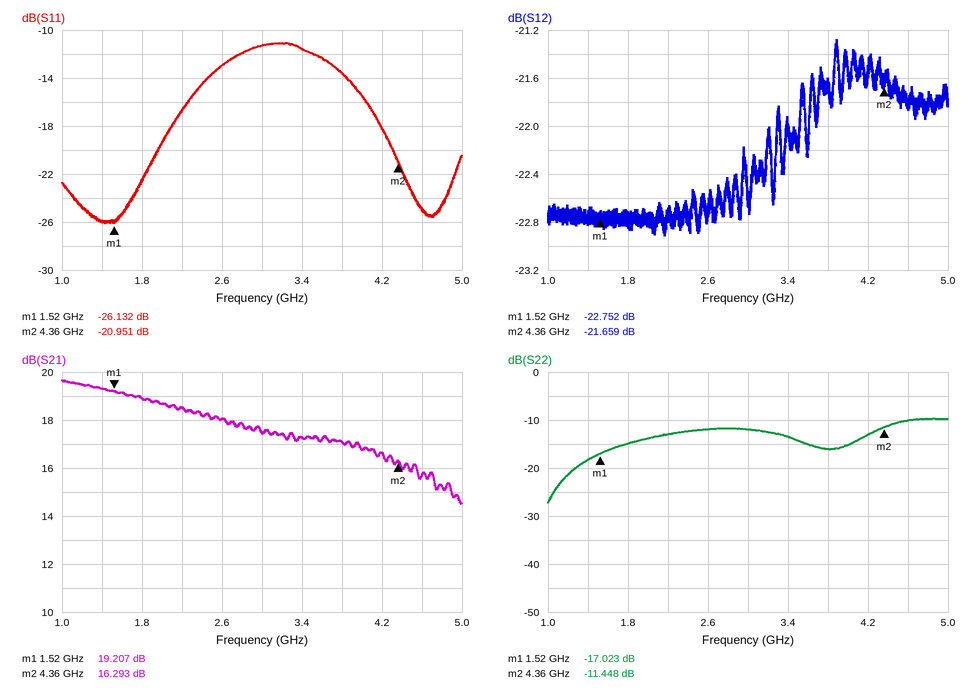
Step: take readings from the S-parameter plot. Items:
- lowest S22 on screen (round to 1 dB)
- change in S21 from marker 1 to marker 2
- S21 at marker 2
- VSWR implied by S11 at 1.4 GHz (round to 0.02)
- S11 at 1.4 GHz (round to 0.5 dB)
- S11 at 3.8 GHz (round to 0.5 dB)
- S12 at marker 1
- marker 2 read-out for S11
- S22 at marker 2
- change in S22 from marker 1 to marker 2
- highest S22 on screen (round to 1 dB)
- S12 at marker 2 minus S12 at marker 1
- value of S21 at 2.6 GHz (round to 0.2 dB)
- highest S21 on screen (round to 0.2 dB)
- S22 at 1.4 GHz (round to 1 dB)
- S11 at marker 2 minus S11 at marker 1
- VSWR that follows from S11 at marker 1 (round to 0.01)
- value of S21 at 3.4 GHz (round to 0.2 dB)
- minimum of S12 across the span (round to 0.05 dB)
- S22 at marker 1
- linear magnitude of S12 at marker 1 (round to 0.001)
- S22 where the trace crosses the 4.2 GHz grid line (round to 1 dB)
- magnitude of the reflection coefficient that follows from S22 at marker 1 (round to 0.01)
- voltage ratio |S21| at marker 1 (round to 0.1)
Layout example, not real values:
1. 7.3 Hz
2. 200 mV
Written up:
1. -27 dB
2. -2.914 dB
3. 16.293 dB
4. 1.10
5. -26.0 dB
6. -13.5 dB
7. -22.752 dB
8. -20.951 dB
9. -11.448 dB
10. 5.575 dB
11. -10 dB
12. 1.093 dB
13. 18.0 dB
14. 19.6 dB
15. -18 dB
16. 5.181 dB
17. 1.10
18. 17.2 dB
19. -22.90 dB
20. -17.023 dB
21. 0.073
22. -13 dB
23. 0.14
24. 9.1
